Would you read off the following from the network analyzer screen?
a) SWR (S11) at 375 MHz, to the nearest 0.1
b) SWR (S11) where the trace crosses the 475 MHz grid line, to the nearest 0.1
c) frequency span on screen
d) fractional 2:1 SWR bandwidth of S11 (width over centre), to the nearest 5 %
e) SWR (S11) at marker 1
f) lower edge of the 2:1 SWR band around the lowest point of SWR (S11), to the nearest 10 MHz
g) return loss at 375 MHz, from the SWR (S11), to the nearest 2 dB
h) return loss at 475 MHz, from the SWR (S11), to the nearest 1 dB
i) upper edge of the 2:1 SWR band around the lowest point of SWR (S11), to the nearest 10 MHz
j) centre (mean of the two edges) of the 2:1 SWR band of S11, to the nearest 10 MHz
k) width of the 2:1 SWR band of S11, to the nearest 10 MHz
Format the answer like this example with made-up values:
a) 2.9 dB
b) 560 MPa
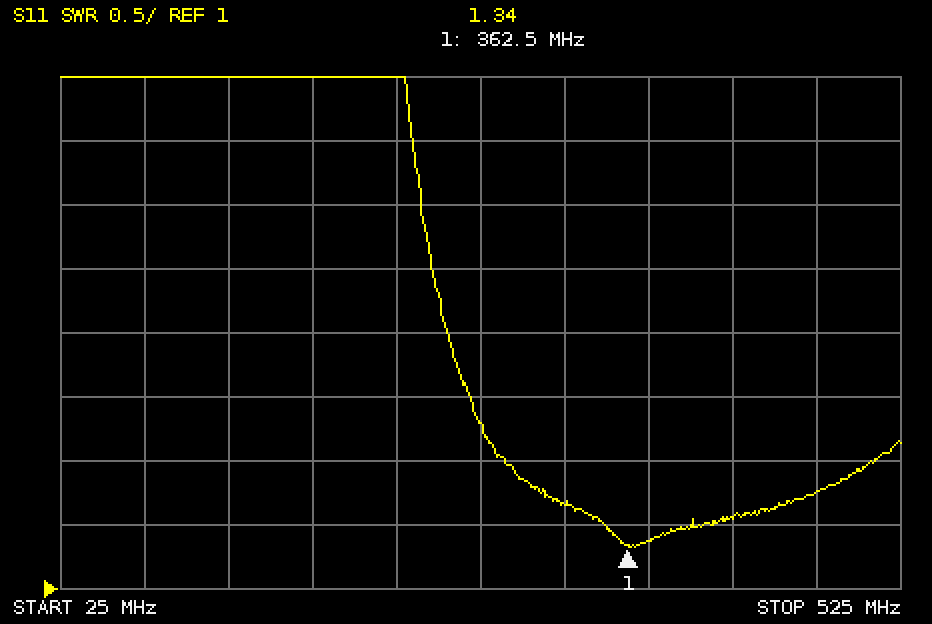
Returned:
a) 1.4
b) 1.8
c) 500 MHz
d) 55 %
e) 1.34
f) 290 MHz
g) 16 dB
h) 11 dB
i) 510 MHz
j) 400 MHz
k) 220 MHz
